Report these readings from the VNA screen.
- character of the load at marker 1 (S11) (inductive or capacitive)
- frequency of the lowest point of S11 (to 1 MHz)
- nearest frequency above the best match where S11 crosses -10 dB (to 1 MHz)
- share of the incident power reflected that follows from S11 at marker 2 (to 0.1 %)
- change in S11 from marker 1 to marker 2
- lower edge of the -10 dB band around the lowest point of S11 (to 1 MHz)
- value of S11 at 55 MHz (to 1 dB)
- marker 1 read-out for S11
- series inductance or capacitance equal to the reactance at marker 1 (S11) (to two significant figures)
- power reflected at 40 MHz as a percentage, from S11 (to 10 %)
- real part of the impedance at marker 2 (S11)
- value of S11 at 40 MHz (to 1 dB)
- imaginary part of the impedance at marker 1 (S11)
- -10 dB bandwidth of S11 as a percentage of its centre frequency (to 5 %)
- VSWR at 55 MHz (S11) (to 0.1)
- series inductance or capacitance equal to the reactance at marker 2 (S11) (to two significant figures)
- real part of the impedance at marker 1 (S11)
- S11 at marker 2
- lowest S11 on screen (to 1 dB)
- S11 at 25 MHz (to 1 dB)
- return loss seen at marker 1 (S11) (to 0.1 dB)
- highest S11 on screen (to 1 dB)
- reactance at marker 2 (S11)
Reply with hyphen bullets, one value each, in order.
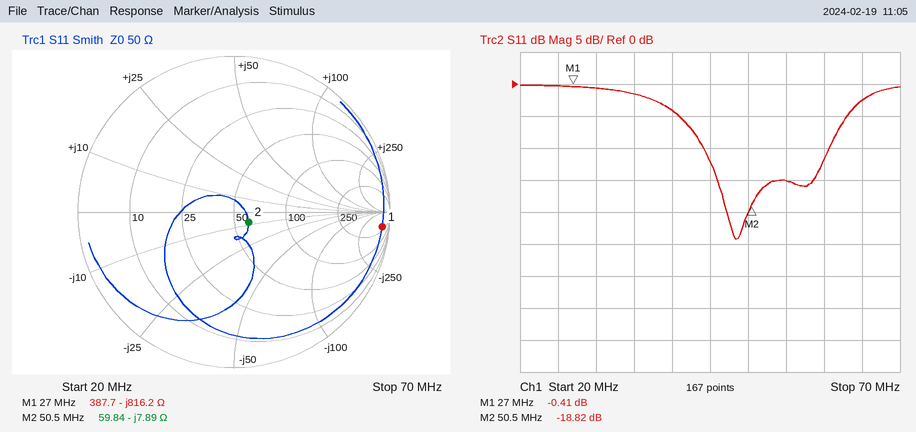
- capacitive
- 48 MHz
- 61 MHz
- 1.3 %
- -18.41 dB
- 44 MHz
- -15 dB
- -0.41 dB
- 7.2 pF
- 40 %
- 59.84 Ω
- -4 dB
- -816.2 Ω
- 30 %
- 1.4
- 400 pF
- 387.7 Ω
- -18.82 dB
- -24 dB
- 0 dB
- 0.4 dB
- 0 dB
- -7.89 Ω
